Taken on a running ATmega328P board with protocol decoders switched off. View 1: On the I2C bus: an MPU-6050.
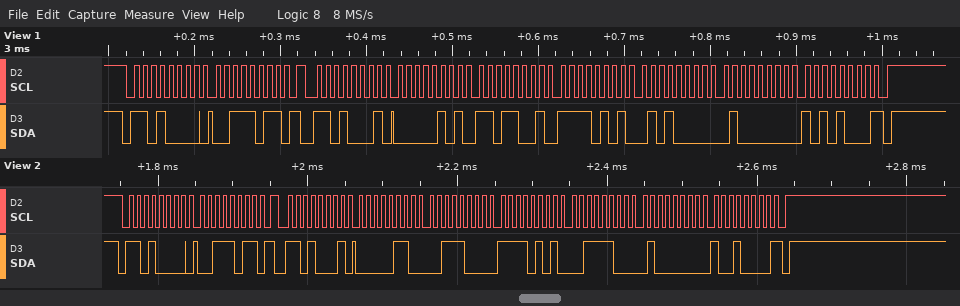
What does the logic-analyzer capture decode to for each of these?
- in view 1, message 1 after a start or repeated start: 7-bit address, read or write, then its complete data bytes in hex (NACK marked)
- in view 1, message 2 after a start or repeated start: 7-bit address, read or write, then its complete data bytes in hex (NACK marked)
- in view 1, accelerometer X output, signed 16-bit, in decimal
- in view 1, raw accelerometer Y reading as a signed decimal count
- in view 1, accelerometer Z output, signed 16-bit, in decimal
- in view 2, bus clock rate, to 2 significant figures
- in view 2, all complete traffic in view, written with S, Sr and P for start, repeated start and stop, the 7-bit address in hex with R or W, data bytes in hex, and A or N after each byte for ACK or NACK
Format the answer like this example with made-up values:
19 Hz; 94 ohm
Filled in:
0x68 write: 3B; 0x68 read: 05 D9 F5 50 40 A8 NACK; 1497; -2736; 16552; 100 kHz; S 68W A 3B A Sr 68R A 06 A 38 A F5 A 3C A 40 A 90 N P
